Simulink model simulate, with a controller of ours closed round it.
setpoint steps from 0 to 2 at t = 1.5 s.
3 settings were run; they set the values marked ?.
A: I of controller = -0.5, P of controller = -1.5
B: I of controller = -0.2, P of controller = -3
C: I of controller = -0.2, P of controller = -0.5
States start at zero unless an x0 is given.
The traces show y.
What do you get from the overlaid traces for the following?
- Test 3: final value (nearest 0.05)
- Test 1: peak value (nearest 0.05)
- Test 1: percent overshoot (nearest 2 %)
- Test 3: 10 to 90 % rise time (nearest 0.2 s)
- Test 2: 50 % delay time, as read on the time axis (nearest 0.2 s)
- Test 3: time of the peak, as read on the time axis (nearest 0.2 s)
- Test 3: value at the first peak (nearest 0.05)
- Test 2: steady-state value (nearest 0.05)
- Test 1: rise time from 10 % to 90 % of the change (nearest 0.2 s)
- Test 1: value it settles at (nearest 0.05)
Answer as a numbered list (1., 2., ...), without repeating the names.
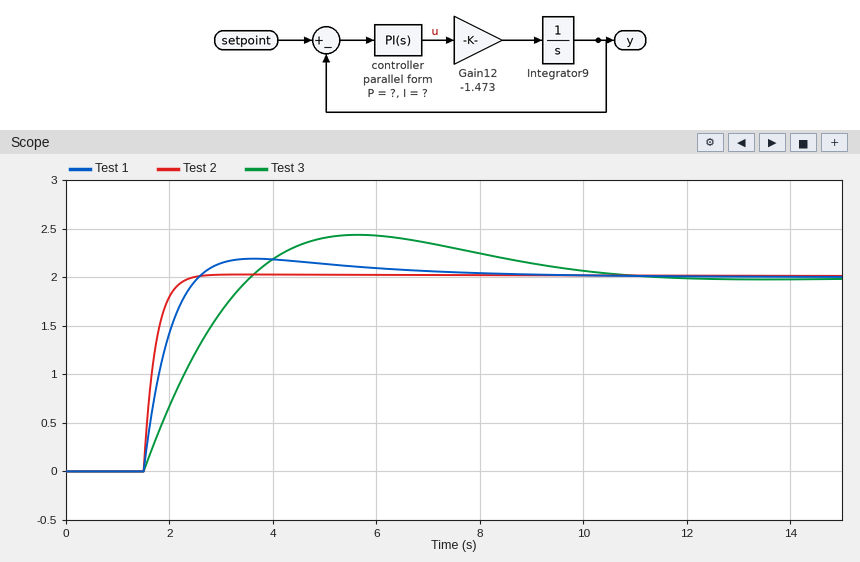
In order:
1. 2.00
2. 2.20
3. 10 %
4. 1.6 s
5. 1.6 s
6. 5.6 s
7. 2.45
8. 2.00
9. 0.8 s
10. 2.00
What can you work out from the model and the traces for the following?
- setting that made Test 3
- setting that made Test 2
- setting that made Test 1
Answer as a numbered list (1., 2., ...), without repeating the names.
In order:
1. C
2. B
3. A
